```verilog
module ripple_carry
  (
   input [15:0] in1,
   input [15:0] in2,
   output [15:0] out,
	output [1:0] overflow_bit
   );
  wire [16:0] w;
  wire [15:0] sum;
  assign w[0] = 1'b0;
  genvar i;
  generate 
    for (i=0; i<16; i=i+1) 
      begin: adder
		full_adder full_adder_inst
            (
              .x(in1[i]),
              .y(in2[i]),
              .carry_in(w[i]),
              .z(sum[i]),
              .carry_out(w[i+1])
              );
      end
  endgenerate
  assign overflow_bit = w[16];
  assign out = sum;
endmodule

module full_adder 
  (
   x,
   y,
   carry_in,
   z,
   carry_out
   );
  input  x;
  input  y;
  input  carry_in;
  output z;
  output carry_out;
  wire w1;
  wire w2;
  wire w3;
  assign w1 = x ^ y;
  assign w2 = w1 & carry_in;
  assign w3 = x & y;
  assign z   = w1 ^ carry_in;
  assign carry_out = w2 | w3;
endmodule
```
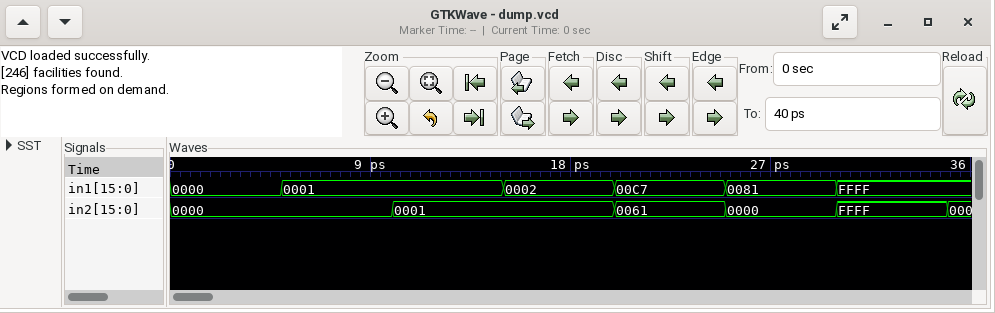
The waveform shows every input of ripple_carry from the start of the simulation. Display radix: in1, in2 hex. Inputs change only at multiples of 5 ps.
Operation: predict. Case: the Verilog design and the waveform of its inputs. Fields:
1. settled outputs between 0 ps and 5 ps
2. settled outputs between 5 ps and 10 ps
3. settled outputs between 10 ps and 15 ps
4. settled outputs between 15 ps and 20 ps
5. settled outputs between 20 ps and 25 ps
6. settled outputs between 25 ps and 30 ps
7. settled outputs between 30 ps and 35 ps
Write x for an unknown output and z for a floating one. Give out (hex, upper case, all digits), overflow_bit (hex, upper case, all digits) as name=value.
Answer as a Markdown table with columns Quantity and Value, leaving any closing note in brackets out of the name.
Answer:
| Quantity | Value |
|---|---|
| settled outputs between 0 ps and 5 ps | out=0000, overflow_bit=0 |
| settled outputs between 5 ps and 10 ps | out=0001, overflow_bit=0 |
| settled outputs between 10 ps and 15 ps | out=0002, overflow_bit=0 |
| settled outputs between 15 ps and 20 ps | out=0003, overflow_bit=0 |
| settled outputs between 20 ps and 25 ps | out=0128, overflow_bit=0 |
| settled outputs between 25 ps and 30 ps | out=0081, overflow_bit=0 |
| settled outputs between 30 ps and 35 ps | out=FFFE, overflow_bit=1 |
